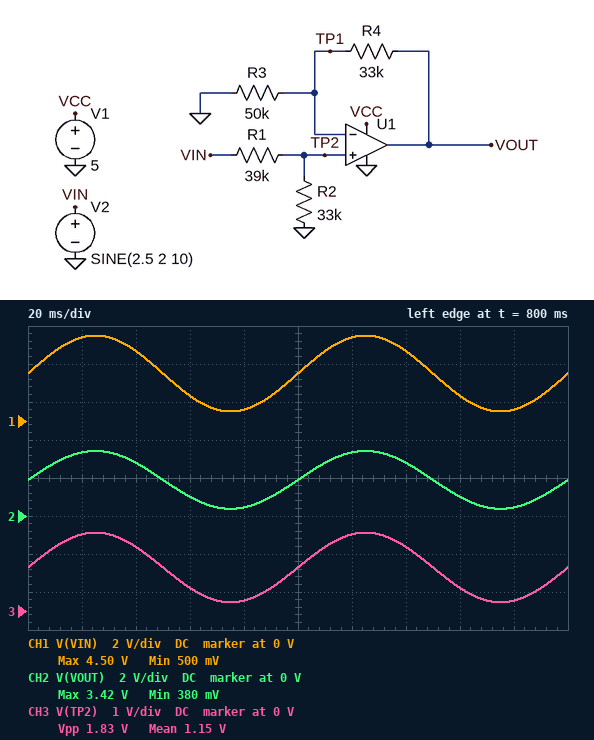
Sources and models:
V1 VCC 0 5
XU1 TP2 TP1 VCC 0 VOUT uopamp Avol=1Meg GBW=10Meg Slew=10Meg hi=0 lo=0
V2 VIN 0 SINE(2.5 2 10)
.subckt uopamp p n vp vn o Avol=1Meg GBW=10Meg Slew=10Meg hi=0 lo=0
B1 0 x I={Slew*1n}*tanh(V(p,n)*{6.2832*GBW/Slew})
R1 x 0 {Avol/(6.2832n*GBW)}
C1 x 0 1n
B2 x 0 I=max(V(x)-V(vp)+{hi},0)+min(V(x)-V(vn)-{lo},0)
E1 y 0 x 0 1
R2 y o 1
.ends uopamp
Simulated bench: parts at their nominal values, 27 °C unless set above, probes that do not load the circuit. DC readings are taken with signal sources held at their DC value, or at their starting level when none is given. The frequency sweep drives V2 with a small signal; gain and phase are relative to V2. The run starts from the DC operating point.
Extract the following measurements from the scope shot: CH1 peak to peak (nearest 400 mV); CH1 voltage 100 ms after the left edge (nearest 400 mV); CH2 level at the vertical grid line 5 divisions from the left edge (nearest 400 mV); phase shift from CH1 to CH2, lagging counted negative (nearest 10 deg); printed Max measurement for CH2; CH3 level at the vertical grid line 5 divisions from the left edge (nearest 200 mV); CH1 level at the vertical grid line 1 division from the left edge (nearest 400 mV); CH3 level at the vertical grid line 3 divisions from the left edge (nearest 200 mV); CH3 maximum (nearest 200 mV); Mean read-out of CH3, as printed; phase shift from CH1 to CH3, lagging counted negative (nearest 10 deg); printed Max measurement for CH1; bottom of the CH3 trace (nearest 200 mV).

4.0 V
2.4 V
2.0 V
0 deg
3.42 V
1.2 V
4.4 V
600 mV
2.0 V
1.15 V
0 deg
4.50 V
200 mV
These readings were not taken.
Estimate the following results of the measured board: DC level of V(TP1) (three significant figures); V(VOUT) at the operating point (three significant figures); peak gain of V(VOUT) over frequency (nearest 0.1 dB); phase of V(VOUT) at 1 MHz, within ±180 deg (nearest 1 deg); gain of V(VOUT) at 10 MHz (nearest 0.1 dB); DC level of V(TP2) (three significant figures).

1.15 V
1.90 V
-2.4 dB
-9 deg
-8.1 dB
1.15 V
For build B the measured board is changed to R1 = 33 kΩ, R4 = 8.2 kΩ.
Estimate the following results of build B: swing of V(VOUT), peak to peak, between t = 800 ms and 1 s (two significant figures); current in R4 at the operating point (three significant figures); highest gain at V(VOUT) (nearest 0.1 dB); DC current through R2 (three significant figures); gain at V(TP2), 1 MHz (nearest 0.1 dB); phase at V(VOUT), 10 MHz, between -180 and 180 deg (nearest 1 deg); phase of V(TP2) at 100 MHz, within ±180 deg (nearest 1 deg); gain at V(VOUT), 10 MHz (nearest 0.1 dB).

2.3 V
25.0 µA
-4.7 dB
37.9 µA
-6.0 dB
-49 deg
0 deg
-8.4 dB
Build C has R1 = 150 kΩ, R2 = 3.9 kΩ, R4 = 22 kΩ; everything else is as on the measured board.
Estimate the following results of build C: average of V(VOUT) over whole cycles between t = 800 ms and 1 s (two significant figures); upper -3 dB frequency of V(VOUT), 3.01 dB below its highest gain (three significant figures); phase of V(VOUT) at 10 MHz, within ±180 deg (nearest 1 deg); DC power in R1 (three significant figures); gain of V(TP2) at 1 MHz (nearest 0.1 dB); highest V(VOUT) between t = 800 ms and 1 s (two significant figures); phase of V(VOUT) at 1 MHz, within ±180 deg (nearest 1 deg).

91 mV
6.94 MHz
-55 deg
39.6 µW
-31.9 dB
160 mV
-8 deg
